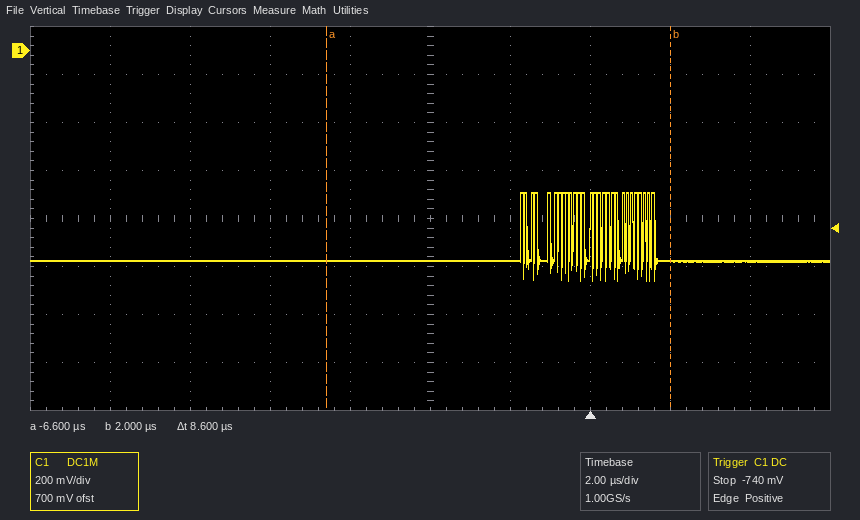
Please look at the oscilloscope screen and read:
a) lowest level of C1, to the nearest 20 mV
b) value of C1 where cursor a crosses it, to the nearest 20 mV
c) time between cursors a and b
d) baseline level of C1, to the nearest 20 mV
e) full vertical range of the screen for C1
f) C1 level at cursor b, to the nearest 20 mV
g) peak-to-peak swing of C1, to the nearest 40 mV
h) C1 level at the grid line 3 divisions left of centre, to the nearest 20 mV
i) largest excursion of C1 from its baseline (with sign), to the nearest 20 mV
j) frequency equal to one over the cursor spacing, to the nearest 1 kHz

-960 mV
-880 mV
8.6 µs
-880 mV
1.6 V
-880 mV
360 mV
-880 mV
+280 mV
116 kHz
